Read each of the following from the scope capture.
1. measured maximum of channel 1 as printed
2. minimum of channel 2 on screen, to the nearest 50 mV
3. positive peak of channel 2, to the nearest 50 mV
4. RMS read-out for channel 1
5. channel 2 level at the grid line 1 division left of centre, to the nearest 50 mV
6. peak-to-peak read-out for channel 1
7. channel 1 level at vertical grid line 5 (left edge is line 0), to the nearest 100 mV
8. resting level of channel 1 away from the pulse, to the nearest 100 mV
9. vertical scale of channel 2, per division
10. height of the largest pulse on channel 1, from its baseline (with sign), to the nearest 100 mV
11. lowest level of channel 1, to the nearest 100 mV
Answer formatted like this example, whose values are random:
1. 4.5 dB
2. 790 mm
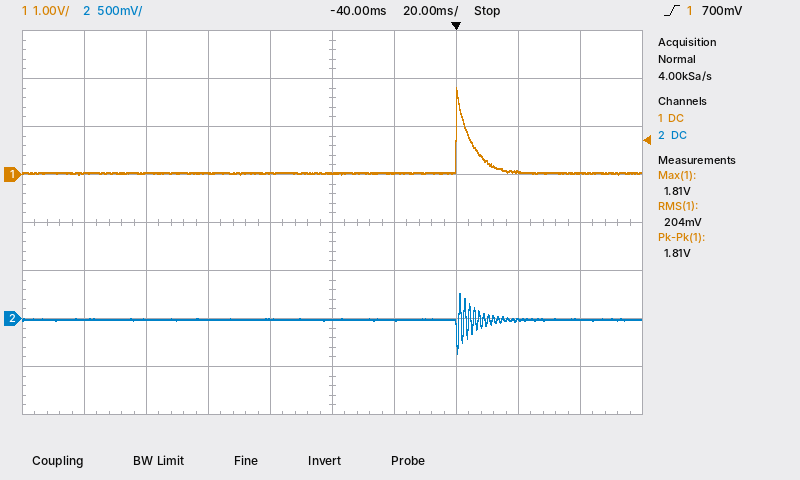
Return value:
1. 1.81 V
2. -350 mV
3. 250 mV
4. 204 mV
5. 0 mV
6. 1.81 V
7. 0.0 V
8. 0.0 V
9. 500 mV
10. +1.8 V
11. 0.0 V
